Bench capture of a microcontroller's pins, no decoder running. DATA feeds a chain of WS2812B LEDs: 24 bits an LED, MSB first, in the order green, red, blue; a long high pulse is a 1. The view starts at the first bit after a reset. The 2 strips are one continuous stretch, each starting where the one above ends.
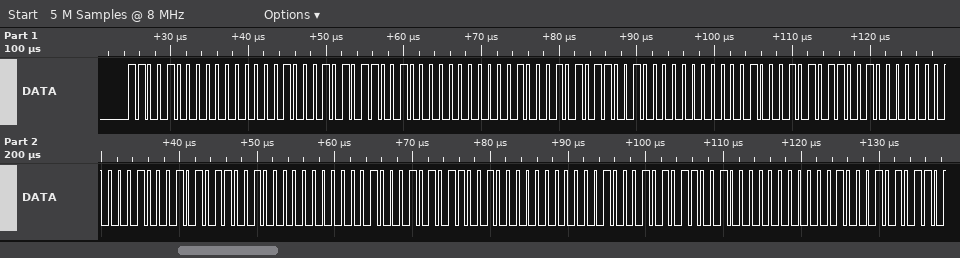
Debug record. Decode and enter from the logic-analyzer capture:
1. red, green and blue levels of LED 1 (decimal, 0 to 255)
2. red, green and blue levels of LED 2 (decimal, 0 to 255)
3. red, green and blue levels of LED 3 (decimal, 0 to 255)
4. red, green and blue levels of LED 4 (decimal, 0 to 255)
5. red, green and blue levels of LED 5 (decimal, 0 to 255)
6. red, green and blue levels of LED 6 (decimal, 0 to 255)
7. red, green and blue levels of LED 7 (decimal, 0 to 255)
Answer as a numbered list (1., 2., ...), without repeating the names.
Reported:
1. 0, 200, 138
2. 0, 200, 138
3. 0, 200, 138
4. 0, 200, 138
5. 0, 200, 138
6. 0, 200, 138
7. 0, 200, 138
